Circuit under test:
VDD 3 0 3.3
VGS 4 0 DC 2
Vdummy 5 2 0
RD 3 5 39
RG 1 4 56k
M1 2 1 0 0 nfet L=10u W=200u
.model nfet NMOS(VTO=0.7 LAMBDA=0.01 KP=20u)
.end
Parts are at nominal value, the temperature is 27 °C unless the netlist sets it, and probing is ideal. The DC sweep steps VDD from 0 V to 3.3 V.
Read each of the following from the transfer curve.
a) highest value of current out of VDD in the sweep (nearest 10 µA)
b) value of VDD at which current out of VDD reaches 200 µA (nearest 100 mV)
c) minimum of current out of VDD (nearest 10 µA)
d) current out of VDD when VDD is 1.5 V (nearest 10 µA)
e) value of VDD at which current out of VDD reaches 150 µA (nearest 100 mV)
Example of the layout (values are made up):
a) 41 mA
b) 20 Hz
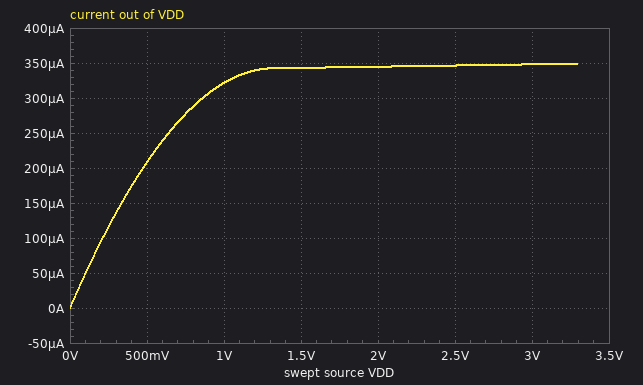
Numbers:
a) 350 µA
b) 500 mV
c) 0 A
d) 340 µA
e) 300 mV
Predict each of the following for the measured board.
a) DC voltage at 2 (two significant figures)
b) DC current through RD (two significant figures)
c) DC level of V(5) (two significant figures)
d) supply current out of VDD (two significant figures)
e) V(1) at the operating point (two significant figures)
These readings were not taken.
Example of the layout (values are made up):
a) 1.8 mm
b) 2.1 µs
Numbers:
a) 3.3 V
b) 350 µA
c) 3.3 V
d) 350 µA
e) 2.0 V
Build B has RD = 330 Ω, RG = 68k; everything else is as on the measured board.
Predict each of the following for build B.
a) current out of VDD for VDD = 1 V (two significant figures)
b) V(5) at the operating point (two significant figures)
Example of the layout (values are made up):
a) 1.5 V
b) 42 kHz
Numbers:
a) 310 µA
b) 3.2 V
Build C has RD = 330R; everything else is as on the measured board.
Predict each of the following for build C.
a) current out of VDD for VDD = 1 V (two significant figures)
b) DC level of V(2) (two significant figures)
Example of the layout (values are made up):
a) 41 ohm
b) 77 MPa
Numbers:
a) 310 µA
b) 3.2 V
